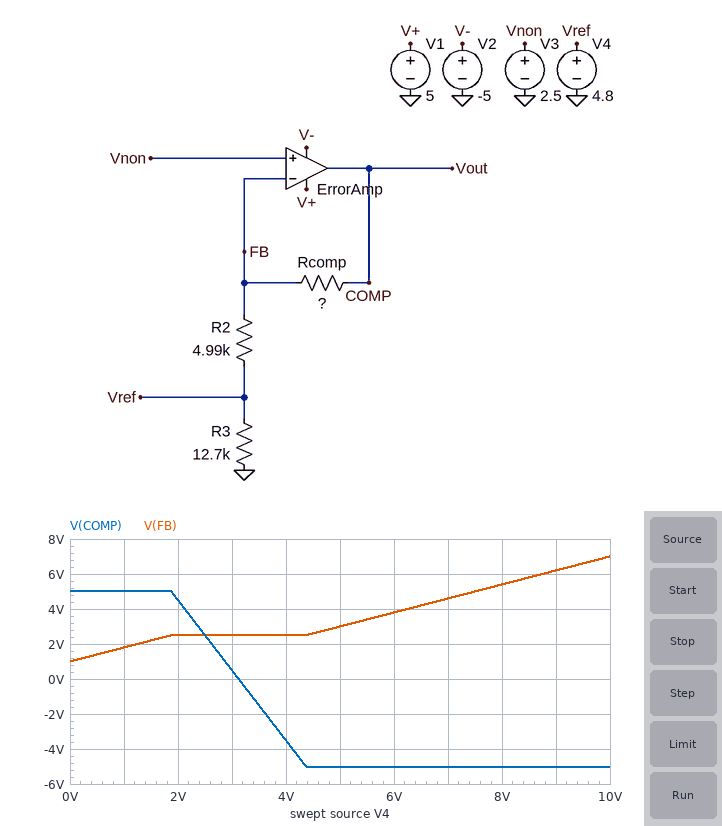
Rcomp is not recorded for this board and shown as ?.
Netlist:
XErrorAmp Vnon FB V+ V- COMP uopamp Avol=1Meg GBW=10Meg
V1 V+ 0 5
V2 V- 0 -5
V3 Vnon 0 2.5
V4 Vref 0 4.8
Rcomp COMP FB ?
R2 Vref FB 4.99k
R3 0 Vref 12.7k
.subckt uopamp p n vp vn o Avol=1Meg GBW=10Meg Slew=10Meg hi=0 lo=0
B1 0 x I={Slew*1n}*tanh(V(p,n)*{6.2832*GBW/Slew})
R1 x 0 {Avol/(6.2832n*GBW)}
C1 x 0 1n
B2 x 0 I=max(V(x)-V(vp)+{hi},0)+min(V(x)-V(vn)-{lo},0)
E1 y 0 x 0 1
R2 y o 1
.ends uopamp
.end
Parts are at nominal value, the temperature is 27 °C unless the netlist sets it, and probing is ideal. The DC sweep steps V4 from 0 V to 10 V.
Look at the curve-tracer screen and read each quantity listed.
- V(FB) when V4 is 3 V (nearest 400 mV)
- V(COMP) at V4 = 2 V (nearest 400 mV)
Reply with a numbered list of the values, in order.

1. 2.4 V
2. 4.4 V
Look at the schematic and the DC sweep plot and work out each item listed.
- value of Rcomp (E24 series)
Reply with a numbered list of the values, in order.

1. 20 kΩ
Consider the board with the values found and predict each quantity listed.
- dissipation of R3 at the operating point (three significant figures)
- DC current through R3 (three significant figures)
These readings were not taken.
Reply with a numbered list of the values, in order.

1. 1.81 mW
2. 378 µA
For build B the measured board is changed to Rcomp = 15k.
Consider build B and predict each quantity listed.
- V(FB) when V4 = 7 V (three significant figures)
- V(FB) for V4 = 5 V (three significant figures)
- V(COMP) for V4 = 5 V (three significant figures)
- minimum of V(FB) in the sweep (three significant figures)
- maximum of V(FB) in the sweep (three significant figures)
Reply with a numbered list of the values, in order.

1. 4.00 V
2. 2.50 V
3. -5.00 V
4. 1.25 V
5. 6.25 V
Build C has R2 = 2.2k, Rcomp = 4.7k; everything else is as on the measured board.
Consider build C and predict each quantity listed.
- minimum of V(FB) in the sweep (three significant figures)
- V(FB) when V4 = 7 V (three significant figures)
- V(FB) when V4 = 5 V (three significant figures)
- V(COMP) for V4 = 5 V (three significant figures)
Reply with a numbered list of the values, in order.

1. 1.60 V
2. 3.17 V
3. 2.50 V
4. -2.84 V
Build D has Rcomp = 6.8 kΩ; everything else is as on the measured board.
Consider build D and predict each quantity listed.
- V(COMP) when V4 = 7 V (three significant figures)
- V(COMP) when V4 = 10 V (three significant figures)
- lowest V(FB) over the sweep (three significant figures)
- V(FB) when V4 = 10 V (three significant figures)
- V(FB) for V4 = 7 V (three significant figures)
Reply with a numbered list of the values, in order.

1. -3.63 V
2. -5.01 V
3. 2.12 V
4. 3.65 V
5. 2.50 V
